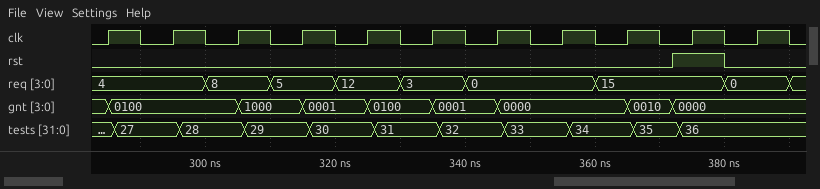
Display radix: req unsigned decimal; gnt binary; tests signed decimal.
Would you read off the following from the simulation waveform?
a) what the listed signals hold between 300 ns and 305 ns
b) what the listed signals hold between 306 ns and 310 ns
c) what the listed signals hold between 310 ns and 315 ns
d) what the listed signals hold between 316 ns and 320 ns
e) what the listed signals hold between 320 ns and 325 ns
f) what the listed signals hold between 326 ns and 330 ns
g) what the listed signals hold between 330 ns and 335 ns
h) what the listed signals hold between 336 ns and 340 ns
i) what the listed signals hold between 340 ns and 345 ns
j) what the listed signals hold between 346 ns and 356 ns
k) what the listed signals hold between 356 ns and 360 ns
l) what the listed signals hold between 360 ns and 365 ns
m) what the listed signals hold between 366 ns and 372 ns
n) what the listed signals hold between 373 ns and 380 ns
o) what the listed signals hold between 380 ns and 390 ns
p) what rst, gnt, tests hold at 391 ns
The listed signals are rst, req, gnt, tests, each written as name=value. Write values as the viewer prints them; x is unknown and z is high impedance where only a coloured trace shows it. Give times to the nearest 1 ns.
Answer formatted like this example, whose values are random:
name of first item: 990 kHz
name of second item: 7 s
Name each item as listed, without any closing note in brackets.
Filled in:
what the listed signals hold between 300 ns and 305 ns: rst=0, req=8, gnt=0100, tests=28
what the listed signals hold between 306 ns and 310 ns: rst=0, req=8, gnt=1000, tests=29
what the listed signals hold between 310 ns and 315 ns: rst=0, req=5, gnt=1000, tests=29
what the listed signals hold between 316 ns and 320 ns: rst=0, req=5, gnt=0001, tests=30
what the listed signals hold between 320 ns and 325 ns: rst=0, req=12, gnt=0001, tests=30
what the listed signals hold between 326 ns and 330 ns: rst=0, req=12, gnt=0100, tests=31
what the listed signals hold between 330 ns and 335 ns: rst=0, req=3, gnt=0100, tests=31
what the listed signals hold between 336 ns and 340 ns: rst=0, req=3, gnt=0001, tests=32
what the listed signals hold between 340 ns and 345 ns: rst=0, req=0, gnt=0001, tests=32
what the listed signals hold between 346 ns and 356 ns: rst=0, req=0, gnt=0000, tests=33
what the listed signals hold between 356 ns and 360 ns: rst=0, req=0, gnt=0000, tests=34
what the listed signals hold between 360 ns and 365 ns: rst=0, req=15, gnt=0000, tests=34
what the listed signals hold between 366 ns and 372 ns: rst=0, req=15, gnt=0010, tests=35
what the listed signals hold between 373 ns and 380 ns: rst=1, req=15, gnt=0000, tests=36
what the listed signals hold between 380 ns and 390 ns: rst=0, req=0, gnt=0000, tests=36
what rst, gnt, tests hold at 391 ns: rst=0, gnt=0000, tests=36
